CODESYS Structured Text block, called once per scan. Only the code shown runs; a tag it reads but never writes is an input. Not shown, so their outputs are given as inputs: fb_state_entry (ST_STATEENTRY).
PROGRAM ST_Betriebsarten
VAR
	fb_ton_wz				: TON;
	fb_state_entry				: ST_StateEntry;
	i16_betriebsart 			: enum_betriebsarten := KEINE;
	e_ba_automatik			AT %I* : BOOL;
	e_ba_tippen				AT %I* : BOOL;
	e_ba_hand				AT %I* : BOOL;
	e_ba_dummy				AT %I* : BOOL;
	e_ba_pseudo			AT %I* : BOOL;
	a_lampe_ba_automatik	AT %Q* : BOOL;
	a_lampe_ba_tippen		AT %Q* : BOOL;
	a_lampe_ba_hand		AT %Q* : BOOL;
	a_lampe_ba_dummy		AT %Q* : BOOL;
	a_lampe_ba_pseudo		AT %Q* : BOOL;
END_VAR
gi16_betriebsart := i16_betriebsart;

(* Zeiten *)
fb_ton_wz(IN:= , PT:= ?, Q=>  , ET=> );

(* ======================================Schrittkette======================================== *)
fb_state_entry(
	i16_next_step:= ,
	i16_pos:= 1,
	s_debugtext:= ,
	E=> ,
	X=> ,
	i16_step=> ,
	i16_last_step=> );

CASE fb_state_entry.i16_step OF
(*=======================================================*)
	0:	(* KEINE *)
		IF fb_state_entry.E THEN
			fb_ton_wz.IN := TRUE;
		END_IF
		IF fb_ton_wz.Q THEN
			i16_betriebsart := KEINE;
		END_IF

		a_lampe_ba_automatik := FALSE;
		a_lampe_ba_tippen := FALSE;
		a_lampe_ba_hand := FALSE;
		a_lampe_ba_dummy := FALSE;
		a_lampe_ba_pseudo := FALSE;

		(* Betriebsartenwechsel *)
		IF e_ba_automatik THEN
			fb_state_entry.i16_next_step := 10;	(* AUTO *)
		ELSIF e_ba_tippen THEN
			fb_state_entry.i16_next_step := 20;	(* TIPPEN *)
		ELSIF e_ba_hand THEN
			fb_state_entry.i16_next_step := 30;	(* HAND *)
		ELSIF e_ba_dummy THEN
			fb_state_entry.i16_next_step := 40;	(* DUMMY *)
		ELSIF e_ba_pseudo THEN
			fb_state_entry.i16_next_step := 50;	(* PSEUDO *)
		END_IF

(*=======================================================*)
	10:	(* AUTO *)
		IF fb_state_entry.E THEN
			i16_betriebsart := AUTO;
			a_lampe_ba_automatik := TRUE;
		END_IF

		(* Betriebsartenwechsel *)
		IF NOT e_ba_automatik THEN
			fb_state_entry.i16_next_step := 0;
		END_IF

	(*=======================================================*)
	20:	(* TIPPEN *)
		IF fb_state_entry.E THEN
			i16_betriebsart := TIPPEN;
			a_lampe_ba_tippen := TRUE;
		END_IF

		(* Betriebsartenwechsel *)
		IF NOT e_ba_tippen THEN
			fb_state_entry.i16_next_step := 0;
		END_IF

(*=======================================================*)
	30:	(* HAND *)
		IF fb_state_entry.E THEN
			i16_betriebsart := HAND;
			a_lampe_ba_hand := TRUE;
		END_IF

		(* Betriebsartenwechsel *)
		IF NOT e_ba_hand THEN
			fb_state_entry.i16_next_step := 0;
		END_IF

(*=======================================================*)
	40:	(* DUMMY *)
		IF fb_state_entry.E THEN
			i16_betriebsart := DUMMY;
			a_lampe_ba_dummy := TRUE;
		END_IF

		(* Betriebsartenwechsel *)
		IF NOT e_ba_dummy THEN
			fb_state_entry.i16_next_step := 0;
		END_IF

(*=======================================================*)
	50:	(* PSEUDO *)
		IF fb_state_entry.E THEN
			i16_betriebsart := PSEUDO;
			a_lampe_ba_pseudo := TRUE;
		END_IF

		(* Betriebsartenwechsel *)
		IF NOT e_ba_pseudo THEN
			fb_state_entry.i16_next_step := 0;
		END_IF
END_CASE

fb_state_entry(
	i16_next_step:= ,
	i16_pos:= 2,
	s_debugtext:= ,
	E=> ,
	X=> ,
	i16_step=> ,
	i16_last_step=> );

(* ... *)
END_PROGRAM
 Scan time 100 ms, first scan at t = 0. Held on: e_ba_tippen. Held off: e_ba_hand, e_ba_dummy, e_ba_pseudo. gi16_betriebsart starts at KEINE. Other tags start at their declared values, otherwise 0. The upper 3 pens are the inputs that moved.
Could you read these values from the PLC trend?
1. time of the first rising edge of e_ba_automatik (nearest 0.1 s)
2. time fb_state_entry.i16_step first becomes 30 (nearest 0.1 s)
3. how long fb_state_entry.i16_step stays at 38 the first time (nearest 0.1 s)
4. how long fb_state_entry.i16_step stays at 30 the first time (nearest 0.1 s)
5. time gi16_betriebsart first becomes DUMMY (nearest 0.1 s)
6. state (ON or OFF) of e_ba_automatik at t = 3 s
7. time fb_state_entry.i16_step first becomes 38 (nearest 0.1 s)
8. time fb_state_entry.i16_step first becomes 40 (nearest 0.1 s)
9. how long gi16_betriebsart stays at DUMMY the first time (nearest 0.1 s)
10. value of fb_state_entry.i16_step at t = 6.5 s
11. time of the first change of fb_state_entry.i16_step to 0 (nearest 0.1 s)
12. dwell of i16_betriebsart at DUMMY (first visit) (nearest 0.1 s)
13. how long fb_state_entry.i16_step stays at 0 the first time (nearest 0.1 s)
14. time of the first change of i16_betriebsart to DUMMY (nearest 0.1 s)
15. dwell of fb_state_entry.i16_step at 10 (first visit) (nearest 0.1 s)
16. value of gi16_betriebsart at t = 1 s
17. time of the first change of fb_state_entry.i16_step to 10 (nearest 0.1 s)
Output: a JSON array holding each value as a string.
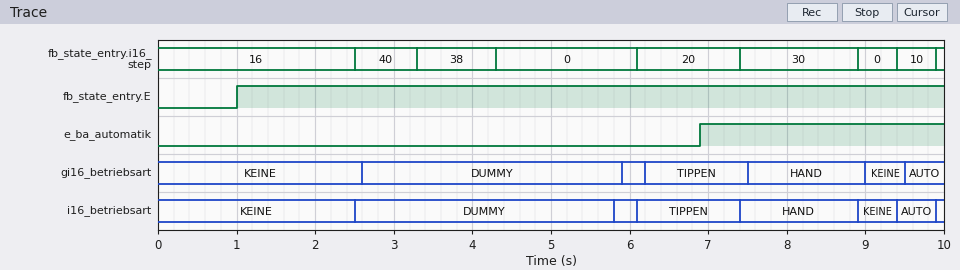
["6.9 s", "7.4 s", "1.0 s", "1.5 s", "2.6 s", "OFF", "3.3 s", "2.5 s", "3.3 s", "20", "4.3 s", "3.3 s", "1.8 s", "2.5 s", "0.5 s", "KEINE", "9.4 s"]
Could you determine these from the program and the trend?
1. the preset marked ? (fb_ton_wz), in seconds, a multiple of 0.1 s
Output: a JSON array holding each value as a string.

["1.4 s"]
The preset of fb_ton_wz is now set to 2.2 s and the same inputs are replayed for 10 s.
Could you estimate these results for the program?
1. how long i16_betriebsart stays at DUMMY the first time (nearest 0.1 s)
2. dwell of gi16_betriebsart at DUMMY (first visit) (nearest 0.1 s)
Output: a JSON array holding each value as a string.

["3.6 s", "3.6 s"]
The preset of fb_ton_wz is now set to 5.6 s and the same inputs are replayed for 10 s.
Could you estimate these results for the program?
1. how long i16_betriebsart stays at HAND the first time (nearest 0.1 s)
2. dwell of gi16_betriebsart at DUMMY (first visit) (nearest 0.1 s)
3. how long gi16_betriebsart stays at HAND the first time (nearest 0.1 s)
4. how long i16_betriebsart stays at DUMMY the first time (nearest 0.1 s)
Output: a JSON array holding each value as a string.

["2.0 s", "3.6 s", "2.0 s", "3.6 s"]
